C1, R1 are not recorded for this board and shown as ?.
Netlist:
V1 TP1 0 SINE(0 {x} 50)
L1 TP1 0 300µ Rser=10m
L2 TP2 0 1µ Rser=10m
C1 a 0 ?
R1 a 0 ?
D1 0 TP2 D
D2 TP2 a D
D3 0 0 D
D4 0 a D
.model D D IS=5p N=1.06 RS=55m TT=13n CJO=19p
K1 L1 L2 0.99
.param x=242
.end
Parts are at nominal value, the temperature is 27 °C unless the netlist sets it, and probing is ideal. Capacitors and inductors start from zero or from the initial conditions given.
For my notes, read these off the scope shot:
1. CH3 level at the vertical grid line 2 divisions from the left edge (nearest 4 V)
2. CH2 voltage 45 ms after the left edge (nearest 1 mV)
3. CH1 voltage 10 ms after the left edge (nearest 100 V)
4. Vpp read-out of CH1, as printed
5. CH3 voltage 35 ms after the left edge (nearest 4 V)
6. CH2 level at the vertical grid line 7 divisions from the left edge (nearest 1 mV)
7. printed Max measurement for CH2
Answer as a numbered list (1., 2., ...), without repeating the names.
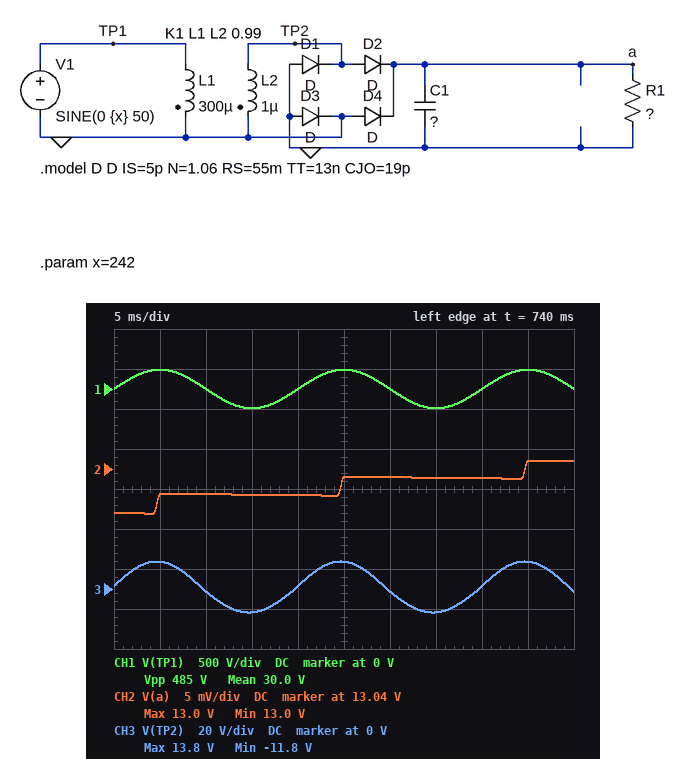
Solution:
1. 0 V
2. 13.046 V
3. 0 V
4. 485 V
5. -12 V
6. 13.044 V
7. 13.0 V
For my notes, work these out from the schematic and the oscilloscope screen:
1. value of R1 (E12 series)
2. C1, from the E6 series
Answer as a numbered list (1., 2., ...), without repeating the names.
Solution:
1. 15 kΩ
2. 68 mF
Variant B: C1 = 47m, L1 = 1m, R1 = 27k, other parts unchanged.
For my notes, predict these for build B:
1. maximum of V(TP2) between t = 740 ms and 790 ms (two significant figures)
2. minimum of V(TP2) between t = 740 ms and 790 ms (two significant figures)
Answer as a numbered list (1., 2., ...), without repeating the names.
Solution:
1. 7.6 V
2. -6.5 V
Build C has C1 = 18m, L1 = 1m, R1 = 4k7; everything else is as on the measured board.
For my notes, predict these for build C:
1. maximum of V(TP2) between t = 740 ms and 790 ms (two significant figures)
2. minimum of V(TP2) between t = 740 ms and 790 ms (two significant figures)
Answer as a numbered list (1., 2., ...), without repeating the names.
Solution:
1. 7.6 V
2. -6.5 V
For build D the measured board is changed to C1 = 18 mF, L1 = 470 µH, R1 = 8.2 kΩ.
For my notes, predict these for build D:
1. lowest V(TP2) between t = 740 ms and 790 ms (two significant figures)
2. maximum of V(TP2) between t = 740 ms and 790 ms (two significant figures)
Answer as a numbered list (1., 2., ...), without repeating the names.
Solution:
1. -9.5 V
2. 11 V
